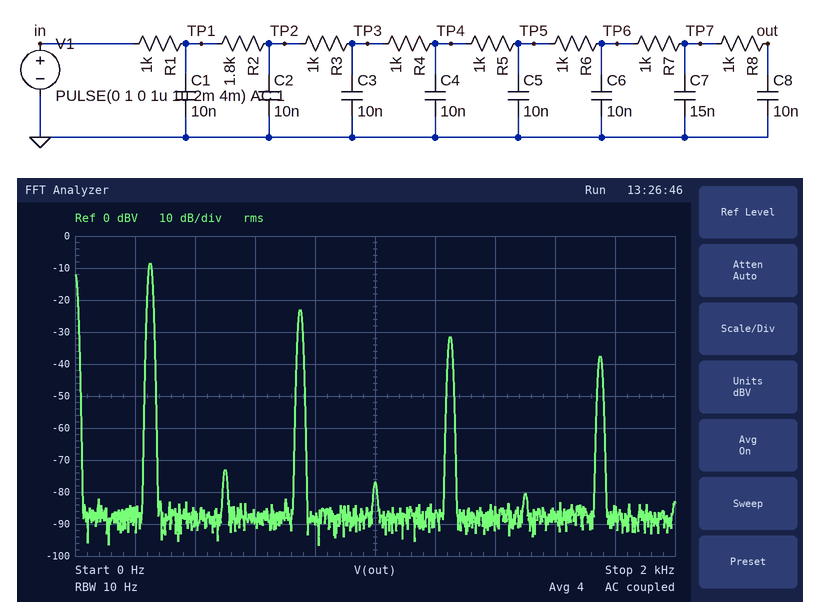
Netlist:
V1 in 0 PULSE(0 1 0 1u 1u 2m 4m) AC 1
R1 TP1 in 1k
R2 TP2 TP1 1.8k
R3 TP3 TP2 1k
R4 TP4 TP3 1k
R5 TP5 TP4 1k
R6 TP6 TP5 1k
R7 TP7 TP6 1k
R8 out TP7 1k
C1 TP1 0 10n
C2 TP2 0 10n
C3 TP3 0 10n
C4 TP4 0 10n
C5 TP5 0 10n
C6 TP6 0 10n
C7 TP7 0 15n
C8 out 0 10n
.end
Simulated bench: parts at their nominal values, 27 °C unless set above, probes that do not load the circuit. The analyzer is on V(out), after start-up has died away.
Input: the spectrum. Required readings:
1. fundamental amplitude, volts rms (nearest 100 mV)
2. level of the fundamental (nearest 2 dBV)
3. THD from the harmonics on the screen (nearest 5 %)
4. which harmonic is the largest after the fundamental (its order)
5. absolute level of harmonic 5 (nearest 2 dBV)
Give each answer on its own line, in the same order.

400 mV
-8 dBV
20 %
3
-32 dBV
